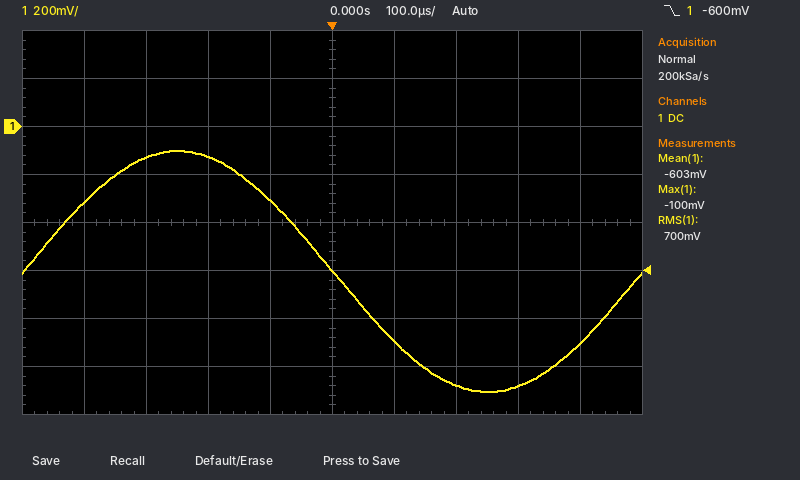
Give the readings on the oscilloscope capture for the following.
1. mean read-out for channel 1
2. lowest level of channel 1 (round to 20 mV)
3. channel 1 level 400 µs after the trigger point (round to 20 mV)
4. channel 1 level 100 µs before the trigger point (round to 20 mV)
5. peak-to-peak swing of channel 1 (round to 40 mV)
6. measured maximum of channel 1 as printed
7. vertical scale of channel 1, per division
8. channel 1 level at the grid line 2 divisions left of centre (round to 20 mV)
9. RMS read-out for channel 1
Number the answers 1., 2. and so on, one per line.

1. -603 mV
2. -1.10 V
3. -900 mV
4. -300 mV
5. 1.00 V
6. -100 mV
7. 200 mV
8. -120 mV
9. 700 mV
